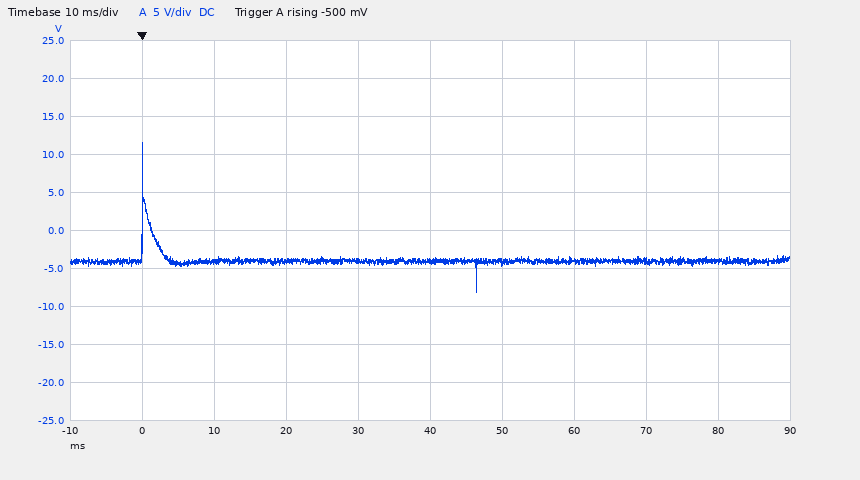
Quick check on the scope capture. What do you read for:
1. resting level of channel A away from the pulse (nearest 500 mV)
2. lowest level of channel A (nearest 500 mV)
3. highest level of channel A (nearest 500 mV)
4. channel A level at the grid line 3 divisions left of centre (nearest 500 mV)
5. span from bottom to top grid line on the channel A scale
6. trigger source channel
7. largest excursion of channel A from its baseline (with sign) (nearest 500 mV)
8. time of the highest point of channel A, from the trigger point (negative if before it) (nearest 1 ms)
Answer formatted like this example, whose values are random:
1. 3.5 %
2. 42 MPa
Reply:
1. -4.0 V
2. -8.0 V
3. 11.5 V
4. -4.0 V
5. 50 V
6. channel A
7. +15.5 V
8. 0 ms
